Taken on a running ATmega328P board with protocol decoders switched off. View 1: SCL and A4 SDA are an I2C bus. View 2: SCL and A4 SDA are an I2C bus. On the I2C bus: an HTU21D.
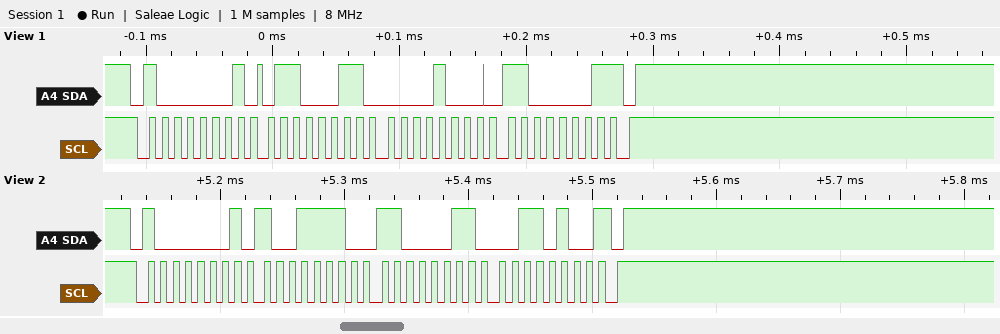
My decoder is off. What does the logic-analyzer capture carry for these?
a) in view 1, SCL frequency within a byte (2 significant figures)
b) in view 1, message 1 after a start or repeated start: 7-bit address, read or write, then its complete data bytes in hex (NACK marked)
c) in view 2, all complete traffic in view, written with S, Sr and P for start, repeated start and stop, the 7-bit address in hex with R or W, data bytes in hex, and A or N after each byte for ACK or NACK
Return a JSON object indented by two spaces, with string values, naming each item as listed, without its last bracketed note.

{
  "in view 1, SCL frequency within a byte": "100 kHz",
  "in view 1, message 1 after a start or repeated start: 7-bit address, read or write, then its complete data bytes in hex": "0x40 read: 63 08 C1 NACK",
  "in view 2, all complete traffic in view, written with S, Sr and P for start, repeated start and stop, the 7-bit address in hex with R or W, data bytes in hex, and A or N after each byte for ACK or NACK": "S 40R A 9E A C3 A 34 N P"
}
